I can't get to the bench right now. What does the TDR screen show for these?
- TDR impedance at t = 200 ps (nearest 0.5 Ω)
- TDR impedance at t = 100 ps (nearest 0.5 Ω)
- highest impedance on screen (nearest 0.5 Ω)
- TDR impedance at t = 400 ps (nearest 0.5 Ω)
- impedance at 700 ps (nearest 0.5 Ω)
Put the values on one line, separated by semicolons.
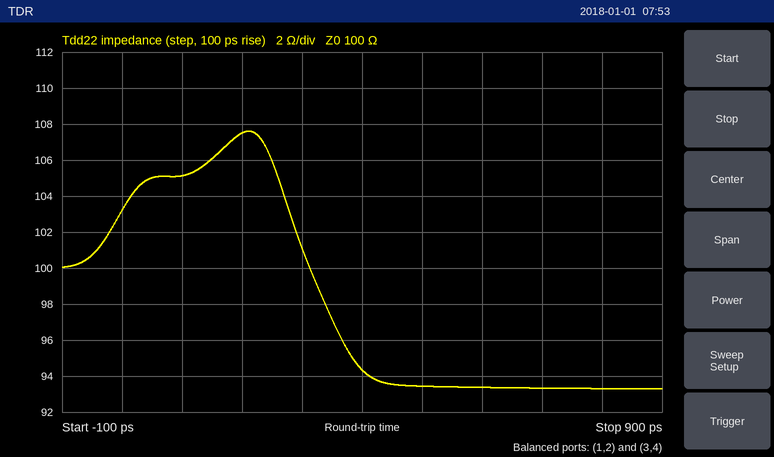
107.5 Ω; 105.0 Ω; 107.5 Ω; 94.5 Ω; 93.5 Ω
